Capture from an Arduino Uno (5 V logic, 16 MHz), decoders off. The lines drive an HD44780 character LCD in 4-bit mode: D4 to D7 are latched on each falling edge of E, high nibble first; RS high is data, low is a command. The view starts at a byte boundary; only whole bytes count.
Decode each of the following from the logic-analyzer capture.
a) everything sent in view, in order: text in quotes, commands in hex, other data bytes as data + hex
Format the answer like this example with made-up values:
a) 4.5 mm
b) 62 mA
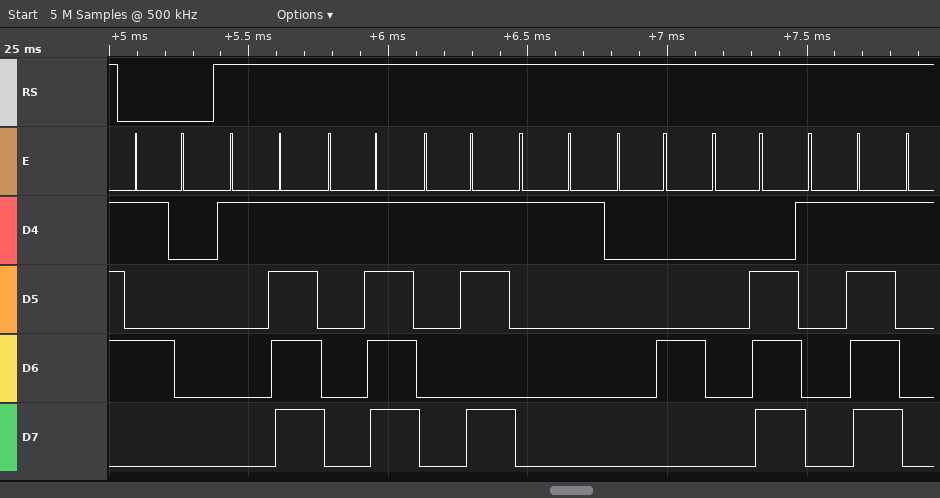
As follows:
a) 0x50 data 1F 1F 1B 11 04 0E 1F
